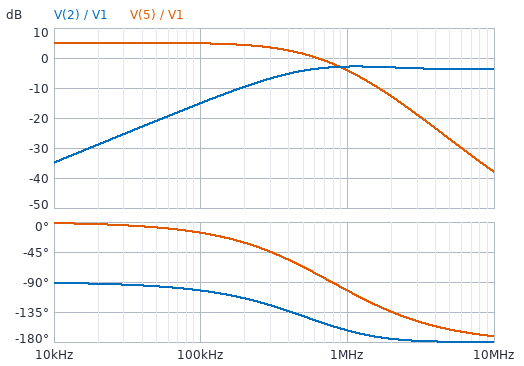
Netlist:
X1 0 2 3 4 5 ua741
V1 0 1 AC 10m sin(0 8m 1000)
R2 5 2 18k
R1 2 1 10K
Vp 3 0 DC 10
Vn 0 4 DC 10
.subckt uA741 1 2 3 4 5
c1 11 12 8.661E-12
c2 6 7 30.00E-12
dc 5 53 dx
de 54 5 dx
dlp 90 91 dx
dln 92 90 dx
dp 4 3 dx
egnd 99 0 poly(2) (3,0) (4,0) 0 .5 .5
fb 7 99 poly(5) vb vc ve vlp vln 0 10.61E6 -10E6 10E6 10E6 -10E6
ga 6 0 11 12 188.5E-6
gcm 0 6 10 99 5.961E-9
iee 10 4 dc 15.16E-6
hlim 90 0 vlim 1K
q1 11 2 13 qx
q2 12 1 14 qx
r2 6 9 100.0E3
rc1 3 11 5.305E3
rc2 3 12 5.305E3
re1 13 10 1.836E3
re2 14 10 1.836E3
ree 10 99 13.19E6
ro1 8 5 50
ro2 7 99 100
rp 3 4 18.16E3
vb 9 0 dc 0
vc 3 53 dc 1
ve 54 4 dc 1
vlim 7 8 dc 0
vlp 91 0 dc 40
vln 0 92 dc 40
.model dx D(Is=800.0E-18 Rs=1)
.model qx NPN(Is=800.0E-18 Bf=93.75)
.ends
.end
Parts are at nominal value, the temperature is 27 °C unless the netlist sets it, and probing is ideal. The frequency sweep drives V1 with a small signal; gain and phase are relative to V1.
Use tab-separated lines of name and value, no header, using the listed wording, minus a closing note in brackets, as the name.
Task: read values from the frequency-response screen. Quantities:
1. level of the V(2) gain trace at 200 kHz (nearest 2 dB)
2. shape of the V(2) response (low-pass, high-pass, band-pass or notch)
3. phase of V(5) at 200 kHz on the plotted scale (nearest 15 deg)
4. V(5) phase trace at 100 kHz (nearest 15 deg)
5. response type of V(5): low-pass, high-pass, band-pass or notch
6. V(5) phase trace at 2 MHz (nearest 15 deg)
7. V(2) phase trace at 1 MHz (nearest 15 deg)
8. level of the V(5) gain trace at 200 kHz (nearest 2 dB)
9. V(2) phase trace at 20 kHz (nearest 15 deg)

level of the V(2) gain trace at 200 kHz	-10 dB
shape of the V(2) response	high-pass
phase of V(5) at 200 kHz on the plotted scale	-30 deg
V(5) phase trace at 100 kHz	-15 deg
response type of V(5): low-pass, high-pass, band-pass or notch	low-pass
V(5) phase trace at 2 MHz	-135 deg
V(2) phase trace at 1 MHz	-165 deg
level of the V(5) gain trace at 200 kHz	4 dB
V(2) phase trace at 20 kHz	-90 deg
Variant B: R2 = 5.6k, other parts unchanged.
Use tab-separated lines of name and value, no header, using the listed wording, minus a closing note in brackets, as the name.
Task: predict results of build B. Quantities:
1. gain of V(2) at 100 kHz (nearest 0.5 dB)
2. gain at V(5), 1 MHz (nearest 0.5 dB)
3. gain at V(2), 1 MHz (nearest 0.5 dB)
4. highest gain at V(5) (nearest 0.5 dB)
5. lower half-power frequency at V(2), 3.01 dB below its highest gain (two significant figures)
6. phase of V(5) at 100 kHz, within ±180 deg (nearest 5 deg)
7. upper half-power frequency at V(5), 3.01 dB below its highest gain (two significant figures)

gain of V(2) at 100 kHz	-25.0 dB
gain at V(5), 1 MHz	-9.0 dB
gain at V(2), 1 MHz	-7.5 dB
highest gain at V(5)	-5.0 dB
lower half-power frequency at V(2), 3.01 dB below its highest gain	600 kHz
phase of V(5) at 100 kHz, within ±180 deg	-10 deg
upper half-power frequency at V(5), 3.01 dB below its highest gain	880 kHz
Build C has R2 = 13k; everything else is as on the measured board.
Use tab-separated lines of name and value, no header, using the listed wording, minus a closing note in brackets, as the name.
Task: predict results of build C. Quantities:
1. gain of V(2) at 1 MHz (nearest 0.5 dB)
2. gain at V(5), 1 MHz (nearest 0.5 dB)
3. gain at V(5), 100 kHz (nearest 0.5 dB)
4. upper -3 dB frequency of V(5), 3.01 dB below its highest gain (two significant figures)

gain of V(2) at 1 MHz	-4.0 dB
gain at V(5), 1 MHz	-5.0 dB
gain at V(5), 100 kHz	2.0 dB
upper -3 dB frequency of V(5), 3.01 dB below its highest gain	550 kHz
